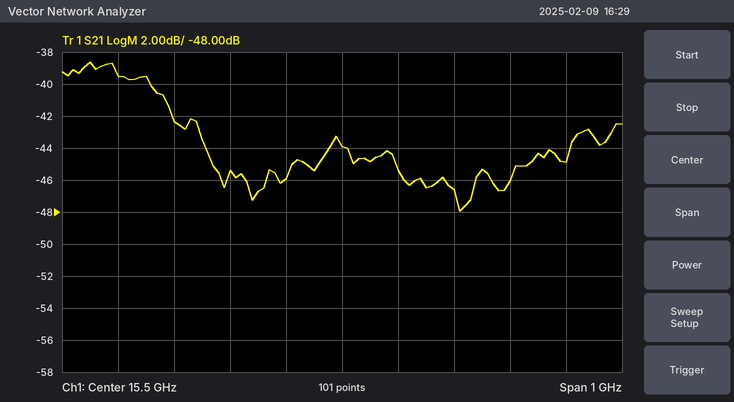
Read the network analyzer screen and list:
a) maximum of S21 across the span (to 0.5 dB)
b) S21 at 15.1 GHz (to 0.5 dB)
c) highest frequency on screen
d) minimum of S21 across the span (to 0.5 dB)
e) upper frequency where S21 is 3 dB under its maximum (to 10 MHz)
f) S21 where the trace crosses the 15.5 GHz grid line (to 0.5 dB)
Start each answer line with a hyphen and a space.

- -38.5 dB
- -39.5 dB
- 16 GHz
- -48.0 dB
- 15.19 GHz
- -44.0 dB
